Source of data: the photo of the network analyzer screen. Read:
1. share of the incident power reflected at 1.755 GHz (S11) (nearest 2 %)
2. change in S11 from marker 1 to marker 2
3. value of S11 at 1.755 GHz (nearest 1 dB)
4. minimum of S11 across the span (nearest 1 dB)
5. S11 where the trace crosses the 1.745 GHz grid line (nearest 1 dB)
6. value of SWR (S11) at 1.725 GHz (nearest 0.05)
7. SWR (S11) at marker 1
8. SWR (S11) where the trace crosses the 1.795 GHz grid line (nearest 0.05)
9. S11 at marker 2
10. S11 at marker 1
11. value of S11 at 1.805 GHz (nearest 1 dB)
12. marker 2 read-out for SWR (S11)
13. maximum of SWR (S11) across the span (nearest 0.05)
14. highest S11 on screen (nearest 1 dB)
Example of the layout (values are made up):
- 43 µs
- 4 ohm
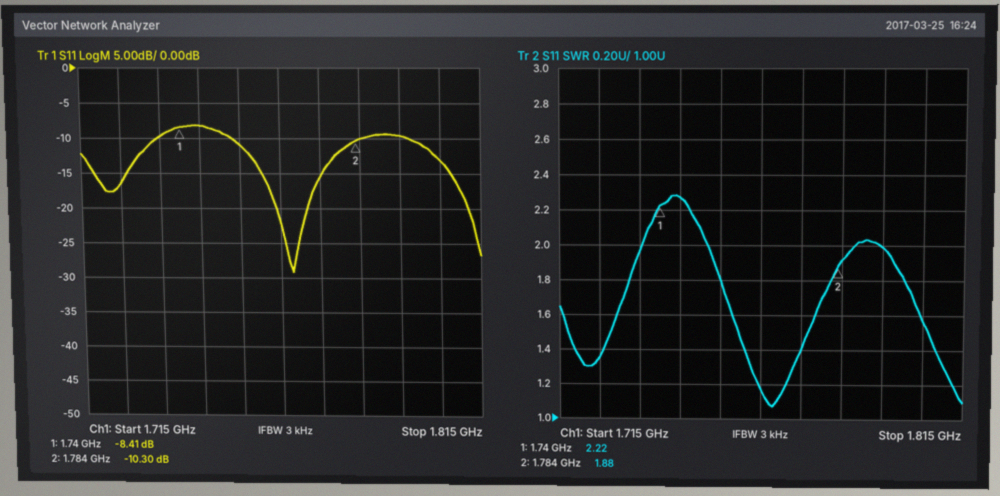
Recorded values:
- 8 %
- -1.89 dB
- -11 dB
- -29 dB
- -8 dB
- 1.35
- 2.22
- 2.00
- -10.30 dB
- -8.41 dB
- -13 dB
- 1.88
- 2.30
- -8 dB
